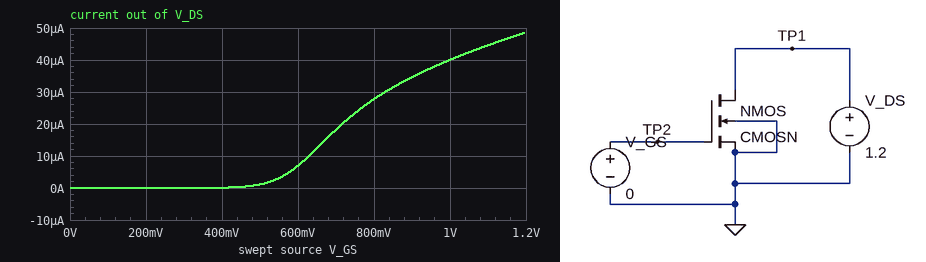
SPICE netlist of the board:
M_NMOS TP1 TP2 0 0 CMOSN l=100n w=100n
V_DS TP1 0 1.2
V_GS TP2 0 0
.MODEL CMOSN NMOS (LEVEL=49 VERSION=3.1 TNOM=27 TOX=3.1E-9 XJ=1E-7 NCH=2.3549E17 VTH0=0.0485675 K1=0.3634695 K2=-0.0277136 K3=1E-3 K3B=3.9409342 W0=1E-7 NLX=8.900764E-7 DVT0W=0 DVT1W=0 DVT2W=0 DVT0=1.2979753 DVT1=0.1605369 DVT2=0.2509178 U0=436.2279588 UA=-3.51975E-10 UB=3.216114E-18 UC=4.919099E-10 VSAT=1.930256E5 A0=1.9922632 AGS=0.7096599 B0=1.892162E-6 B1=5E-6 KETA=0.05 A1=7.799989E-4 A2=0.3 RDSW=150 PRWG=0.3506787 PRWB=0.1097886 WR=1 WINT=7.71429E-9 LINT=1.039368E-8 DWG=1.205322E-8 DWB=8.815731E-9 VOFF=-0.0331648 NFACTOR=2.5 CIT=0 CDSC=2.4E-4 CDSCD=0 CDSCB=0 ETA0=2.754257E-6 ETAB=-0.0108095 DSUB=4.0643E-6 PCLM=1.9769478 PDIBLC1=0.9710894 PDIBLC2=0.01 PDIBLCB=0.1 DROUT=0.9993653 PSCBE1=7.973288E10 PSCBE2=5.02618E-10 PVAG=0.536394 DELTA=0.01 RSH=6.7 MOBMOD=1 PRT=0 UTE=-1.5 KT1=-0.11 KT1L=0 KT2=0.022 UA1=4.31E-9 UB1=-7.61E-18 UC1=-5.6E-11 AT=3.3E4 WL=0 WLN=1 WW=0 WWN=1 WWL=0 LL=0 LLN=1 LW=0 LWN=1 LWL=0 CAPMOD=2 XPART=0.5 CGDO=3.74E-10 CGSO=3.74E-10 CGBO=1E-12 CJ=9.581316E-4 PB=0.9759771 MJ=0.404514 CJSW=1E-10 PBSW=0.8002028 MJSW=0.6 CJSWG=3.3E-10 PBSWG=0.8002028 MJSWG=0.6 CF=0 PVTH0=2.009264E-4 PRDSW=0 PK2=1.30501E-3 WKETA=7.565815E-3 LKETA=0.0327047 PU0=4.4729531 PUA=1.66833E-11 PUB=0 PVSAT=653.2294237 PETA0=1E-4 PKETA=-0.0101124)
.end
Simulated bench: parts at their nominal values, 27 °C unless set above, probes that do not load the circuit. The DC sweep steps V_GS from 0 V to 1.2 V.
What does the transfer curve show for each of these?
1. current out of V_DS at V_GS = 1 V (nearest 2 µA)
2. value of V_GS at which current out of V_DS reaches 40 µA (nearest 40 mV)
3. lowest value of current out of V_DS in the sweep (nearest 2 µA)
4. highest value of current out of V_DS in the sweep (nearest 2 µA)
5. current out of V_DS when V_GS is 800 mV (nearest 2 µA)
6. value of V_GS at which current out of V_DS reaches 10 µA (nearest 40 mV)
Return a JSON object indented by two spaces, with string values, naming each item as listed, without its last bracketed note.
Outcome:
{
  "current out of V_DS at V_GS = 1 V": "40 µA",
  "value of V_GS at which current out of V_DS reaches 40 µA": "1.00 V",
  "lowest value of current out of V_DS in the sweep": "0 A",
  "highest value of current out of V_DS in the sweep": "48 µA",
  "current out of V_DS when V_GS is 800 mV": "28 µA",
  "value of V_GS at which current out of V_DS reaches 10 µA": "640 mV"
}
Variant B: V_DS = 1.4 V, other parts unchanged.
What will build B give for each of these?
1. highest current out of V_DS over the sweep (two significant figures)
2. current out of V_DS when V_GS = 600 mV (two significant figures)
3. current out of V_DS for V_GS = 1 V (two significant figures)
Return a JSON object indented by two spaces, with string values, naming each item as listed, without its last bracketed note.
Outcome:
{
  "highest current out of V_DS over the sweep": "51 µA",
  "current out of V_DS when V_GS = 600 mV": "8.9 µA",
  "current out of V_DS for V_GS = 1 V": "43 µA"
}
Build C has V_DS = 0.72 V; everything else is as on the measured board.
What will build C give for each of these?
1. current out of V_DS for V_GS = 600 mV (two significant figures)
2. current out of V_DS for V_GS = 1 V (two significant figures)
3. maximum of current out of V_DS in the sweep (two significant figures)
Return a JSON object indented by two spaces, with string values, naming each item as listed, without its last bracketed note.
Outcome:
{
  "current out of V_DS for V_GS = 600 mV": "3.4 µA",
  "current out of V_DS for V_GS = 1 V": "33 µA",
  "maximum of current out of V_DS in the sweep": "41 µA"
}
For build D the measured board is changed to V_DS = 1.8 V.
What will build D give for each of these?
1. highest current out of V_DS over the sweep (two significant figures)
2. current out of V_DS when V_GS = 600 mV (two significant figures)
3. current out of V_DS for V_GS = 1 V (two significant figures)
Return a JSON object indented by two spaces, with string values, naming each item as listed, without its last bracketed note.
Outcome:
{
  "highest current out of V_DS over the sweep": "57 µA",
  "current out of V_DS when V_GS = 600 mV": "14 µA",
  "current out of V_DS for V_GS = 1 V": "49 µA"
}
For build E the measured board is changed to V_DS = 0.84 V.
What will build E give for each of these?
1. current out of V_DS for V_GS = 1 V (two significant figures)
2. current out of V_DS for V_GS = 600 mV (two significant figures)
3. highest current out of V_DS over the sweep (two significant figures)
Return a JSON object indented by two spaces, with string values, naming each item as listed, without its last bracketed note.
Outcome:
{
  "current out of V_DS for V_GS = 1 V": "35 µA",
  "current out of V_DS for V_GS = 600 mV": "4.1 µA",
  "highest current out of V_DS over the sweep": "43 µA"
}
